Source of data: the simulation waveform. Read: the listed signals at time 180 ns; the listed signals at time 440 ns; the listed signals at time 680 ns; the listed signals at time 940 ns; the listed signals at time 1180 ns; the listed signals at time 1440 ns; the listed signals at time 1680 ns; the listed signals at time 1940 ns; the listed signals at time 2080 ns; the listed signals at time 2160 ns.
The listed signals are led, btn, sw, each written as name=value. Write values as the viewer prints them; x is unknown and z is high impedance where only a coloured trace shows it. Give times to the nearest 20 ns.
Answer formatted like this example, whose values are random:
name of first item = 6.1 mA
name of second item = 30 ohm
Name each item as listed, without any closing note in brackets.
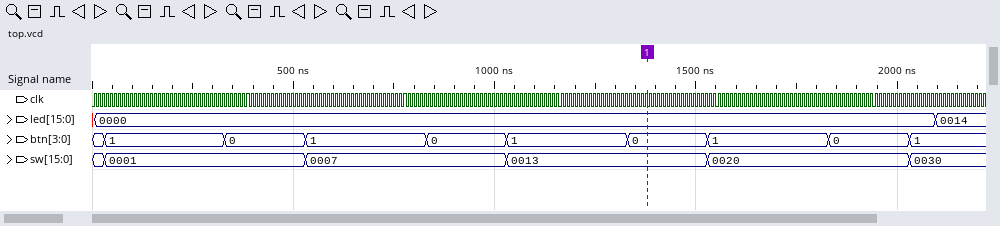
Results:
the listed signals at time 180 ns = led=0000, btn=1, sw=0001
the listed signals at time 440 ns = led=0000, btn=0, sw=0001
the listed signals at time 680 ns = led=0000, btn=1, sw=0007
the listed signals at time 940 ns = led=0000, btn=0, sw=0007
the listed signals at time 1180 ns = led=0000, btn=1, sw=0013
the listed signals at time 1440 ns = led=0000, btn=0, sw=0013
the listed signals at time 1680 ns = led=0000, btn=1, sw=0020
the listed signals at time 1940 ns = led=0000, btn=0, sw=0020
the listed signals at time 2080 ns = led=0000, btn=1, sw=0030
the listed signals at time 2160 ns = led=0014, btn=1, sw=0030
